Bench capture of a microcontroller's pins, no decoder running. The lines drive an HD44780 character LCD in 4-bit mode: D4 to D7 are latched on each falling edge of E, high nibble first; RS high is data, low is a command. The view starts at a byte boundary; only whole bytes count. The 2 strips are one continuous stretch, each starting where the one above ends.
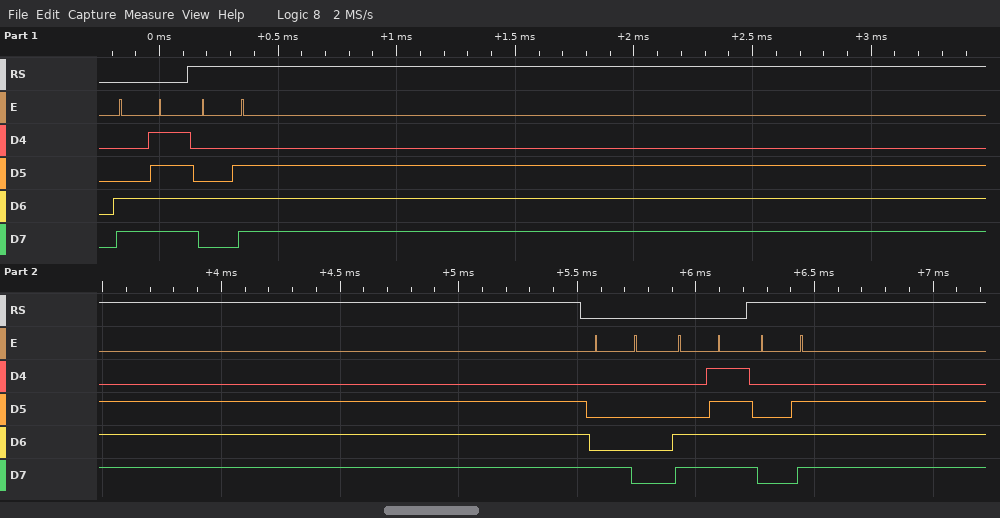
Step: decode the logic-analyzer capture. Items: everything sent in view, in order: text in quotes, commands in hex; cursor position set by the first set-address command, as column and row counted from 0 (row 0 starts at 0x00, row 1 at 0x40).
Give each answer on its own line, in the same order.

0xCF "N" 0x80 0xCF "N"
column 15, row 1
